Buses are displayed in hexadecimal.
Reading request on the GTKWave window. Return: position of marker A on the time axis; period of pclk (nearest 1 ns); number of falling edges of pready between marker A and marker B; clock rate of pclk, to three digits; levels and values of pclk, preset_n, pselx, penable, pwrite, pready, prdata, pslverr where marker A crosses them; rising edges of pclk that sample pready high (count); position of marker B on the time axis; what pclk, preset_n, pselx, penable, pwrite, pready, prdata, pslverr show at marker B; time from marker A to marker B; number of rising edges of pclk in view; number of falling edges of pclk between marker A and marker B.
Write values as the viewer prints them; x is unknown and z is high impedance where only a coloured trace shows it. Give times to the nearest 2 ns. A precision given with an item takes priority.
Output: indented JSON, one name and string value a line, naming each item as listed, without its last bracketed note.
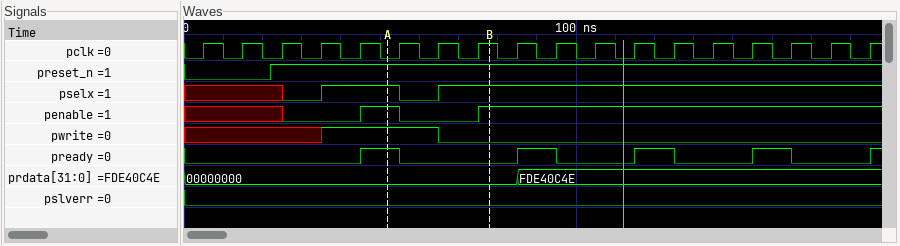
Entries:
{
  "position of marker A on the time axis": "52 ns",
  "period of pclk": "10 ns",
  "number of falling edges of pready between marker A and marker B": "1",
  "clock rate of pclk, to three digits": "100 MHz",
  "levels and values of pclk, preset_n, pselx, penable, pwrite, pready, prdata, pslverr where marker A crosses them": "pclk=0, preset_n=1, pselx=1, penable=1, pwrite=1, pready=1, prdata=00000000, pslverr=0",
  "rising edges of pclk that sample pready high": "4",
  "position of marker B on the time axis": "78 ns",
  "what pclk, preset_n, pselx, penable, pwrite, pready, prdata, pslverr show at marker B": "pclk=1, preset_n=1, pselx=1, penable=1, pwrite=0, pready=0, prdata=00000000, pslverr=0",
  "time from marker A to marker B": "26 ns",
  "number of rising edges of pclk in view": "18",
  "number of falling edges of pclk between marker A and marker B": "2"
}
